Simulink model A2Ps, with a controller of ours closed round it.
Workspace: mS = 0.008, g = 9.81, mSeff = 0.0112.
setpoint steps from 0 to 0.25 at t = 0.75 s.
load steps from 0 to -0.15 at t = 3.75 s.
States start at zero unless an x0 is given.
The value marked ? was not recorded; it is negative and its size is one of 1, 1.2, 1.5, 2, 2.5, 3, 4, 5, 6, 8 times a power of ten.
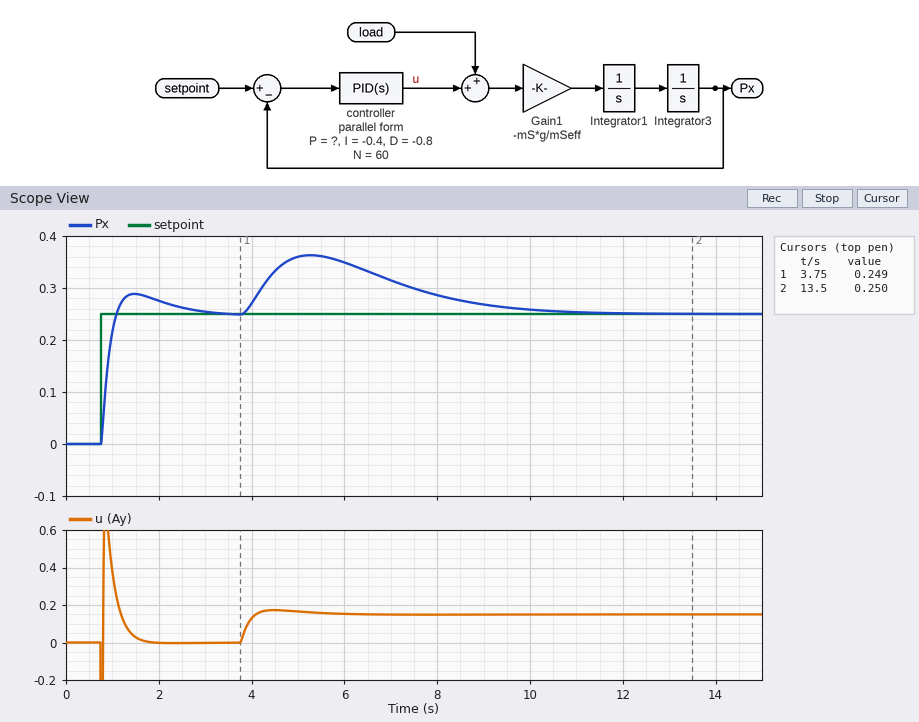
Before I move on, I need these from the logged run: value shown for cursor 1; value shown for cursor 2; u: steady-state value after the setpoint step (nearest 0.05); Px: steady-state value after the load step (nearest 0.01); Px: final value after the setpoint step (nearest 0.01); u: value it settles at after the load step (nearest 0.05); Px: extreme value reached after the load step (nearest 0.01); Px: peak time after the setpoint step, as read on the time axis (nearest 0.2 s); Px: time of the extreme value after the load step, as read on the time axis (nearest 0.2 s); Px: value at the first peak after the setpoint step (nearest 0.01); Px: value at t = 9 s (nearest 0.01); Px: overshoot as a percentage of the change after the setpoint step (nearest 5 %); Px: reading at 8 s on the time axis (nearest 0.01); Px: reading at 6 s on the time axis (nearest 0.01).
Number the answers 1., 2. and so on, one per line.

1. 0.249
2. 0.250
3. 0.00
4. 0.25
5. 0.25
6. 0.15
7. 0.36
8. 1.4 s
9. 5.2 s
10. 0.29
11. 0.27
12. 15 %
13. 0.29
14. 0.35
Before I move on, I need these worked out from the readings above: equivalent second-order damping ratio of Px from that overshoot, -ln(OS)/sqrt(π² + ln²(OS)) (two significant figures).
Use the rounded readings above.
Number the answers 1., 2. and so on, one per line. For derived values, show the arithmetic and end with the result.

1. ln(0.15) = -1.897; 1.897 / sqrt(9.870 + 3.599) = 0.52
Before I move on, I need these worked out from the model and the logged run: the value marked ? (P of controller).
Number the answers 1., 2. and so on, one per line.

1. -1
